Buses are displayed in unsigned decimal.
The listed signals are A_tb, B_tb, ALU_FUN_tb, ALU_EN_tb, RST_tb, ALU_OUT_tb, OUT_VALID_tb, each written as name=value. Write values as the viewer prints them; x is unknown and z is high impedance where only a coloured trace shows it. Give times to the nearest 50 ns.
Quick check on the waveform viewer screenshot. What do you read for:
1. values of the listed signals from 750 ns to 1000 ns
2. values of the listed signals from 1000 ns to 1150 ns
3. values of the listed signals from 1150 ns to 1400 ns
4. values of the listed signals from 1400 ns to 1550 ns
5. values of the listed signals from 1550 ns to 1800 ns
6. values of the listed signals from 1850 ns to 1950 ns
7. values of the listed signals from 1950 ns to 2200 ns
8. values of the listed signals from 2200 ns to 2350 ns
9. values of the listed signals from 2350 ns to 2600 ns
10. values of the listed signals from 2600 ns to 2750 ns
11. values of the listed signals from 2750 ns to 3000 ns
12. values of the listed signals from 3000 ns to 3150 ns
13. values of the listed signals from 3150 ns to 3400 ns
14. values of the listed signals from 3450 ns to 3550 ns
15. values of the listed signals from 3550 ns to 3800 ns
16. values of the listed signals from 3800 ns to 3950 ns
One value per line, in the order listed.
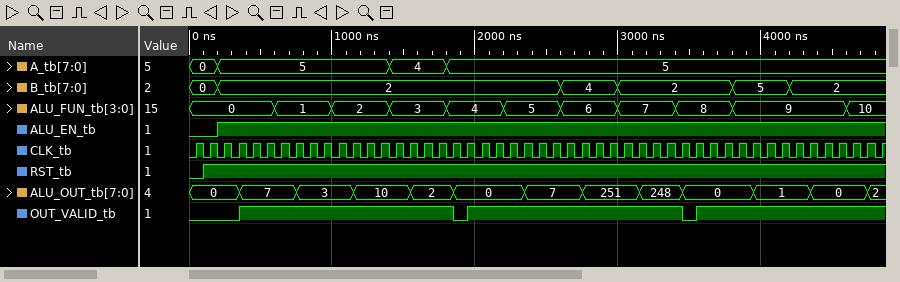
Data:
A_tb=5, B_tb=2, ALU_FUN_tb=1, ALU_EN_tb=1, RST_tb=1, ALU_OUT_tb=3, OUT_VALID_tb=1
A_tb=5, B_tb=2, ALU_FUN_tb=2, ALU_EN_tb=1, RST_tb=1, ALU_OUT_tb=3, OUT_VALID_tb=1
A_tb=5, B_tb=2, ALU_FUN_tb=2, ALU_EN_tb=1, RST_tb=1, ALU_OUT_tb=10, OUT_VALID_tb=1
A_tb=4, B_tb=2, ALU_FUN_tb=3, ALU_EN_tb=1, RST_tb=1, ALU_OUT_tb=10, OUT_VALID_tb=1
A_tb=4, B_tb=2, ALU_FUN_tb=3, ALU_EN_tb=1, RST_tb=1, ALU_OUT_tb=2, OUT_VALID_tb=1
A_tb=5, B_tb=2, ALU_FUN_tb=4, ALU_EN_tb=1, RST_tb=1, ALU_OUT_tb=0, OUT_VALID_tb=0
A_tb=5, B_tb=2, ALU_FUN_tb=4, ALU_EN_tb=1, RST_tb=1, ALU_OUT_tb=0, OUT_VALID_tb=1
A_tb=5, B_tb=2, ALU_FUN_tb=5, ALU_EN_tb=1, RST_tb=1, ALU_OUT_tb=0, OUT_VALID_tb=1
A_tb=5, B_tb=2, ALU_FUN_tb=5, ALU_EN_tb=1, RST_tb=1, ALU_OUT_tb=7, OUT_VALID_tb=1
A_tb=5, B_tb=4, ALU_FUN_tb=6, ALU_EN_tb=1, RST_tb=1, ALU_OUT_tb=7, OUT_VALID_tb=1
A_tb=5, B_tb=4, ALU_FUN_tb=6, ALU_EN_tb=1, RST_tb=1, ALU_OUT_tb=251, OUT_VALID_tb=1
A_tb=5, B_tb=2, ALU_FUN_tb=7, ALU_EN_tb=1, RST_tb=1, ALU_OUT_tb=251, OUT_VALID_tb=1
A_tb=5, B_tb=2, ALU_FUN_tb=7, ALU_EN_tb=1, RST_tb=1, ALU_OUT_tb=248, OUT_VALID_tb=1
A_tb=5, B_tb=2, ALU_FUN_tb=8, ALU_EN_tb=1, RST_tb=1, ALU_OUT_tb=0, OUT_VALID_tb=0
A_tb=5, B_tb=2, ALU_FUN_tb=8, ALU_EN_tb=1, RST_tb=1, ALU_OUT_tb=0, OUT_VALID_tb=1
A_tb=5, B_tb=5, ALU_FUN_tb=9, ALU_EN_tb=1, RST_tb=1, ALU_OUT_tb=0, OUT_VALID_tb=1
